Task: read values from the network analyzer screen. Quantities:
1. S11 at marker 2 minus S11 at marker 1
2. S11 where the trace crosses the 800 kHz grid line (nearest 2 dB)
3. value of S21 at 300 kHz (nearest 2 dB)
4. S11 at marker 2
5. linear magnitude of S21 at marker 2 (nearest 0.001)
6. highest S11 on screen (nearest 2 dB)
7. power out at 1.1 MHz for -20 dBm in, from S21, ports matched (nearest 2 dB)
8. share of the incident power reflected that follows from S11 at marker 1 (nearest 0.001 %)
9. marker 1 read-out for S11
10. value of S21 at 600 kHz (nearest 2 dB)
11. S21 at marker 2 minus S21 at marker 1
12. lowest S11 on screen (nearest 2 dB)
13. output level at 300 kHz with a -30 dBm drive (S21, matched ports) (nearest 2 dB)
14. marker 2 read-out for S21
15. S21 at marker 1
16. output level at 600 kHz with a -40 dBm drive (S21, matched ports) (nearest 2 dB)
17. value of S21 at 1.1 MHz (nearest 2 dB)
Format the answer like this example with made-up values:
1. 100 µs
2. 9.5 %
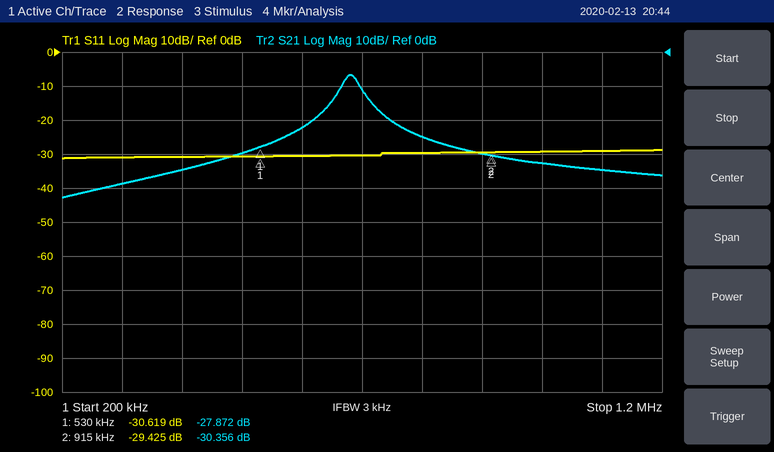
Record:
1. 1.194 dB
2. -30 dB
3. -38 dB
4. -29.425 dB
5. 0.030
6. -28 dB
7. -54 dBm
8. 0.087 %
9. -30.619 dB
10. -22 dB
11. -2.484 dB
12. -32 dB
13. -68 dBm
14. -30.356 dB
15. -27.872 dB
16. -62 dBm
17. -34 dB
